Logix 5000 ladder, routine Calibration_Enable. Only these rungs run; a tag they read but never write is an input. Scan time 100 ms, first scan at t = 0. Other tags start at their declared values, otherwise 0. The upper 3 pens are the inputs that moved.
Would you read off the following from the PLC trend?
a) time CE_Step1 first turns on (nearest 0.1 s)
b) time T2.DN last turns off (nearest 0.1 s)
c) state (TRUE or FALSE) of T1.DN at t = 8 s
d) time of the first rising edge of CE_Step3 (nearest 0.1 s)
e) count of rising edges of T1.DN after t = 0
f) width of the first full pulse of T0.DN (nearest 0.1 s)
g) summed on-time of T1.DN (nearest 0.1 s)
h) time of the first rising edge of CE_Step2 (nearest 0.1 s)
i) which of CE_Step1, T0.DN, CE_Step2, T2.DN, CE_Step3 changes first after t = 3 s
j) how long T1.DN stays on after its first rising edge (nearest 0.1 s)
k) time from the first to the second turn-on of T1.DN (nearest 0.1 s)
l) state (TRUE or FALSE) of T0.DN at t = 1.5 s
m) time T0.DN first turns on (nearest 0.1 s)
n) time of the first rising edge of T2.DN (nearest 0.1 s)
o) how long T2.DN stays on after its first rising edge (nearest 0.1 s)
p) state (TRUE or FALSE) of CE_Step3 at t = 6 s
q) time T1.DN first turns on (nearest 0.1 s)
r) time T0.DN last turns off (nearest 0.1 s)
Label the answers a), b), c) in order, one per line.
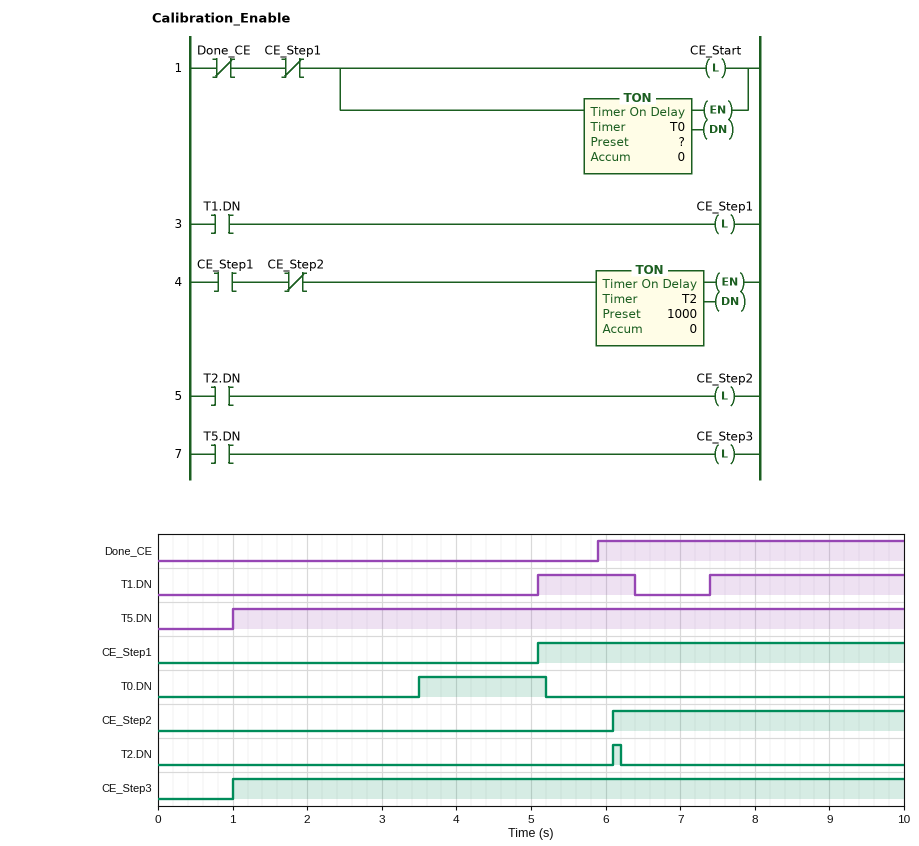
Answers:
a) 5.1 s
b) 6.2 s
c) TRUE
d) 1.0 s
e) 2
f) 1.7 s
g) 3.9 s
h) 6.1 s
i) T0.DN
j) 1.3 s
k) 2.3 s
l) FALSE
m) 3.5 s
n) 6.1 s
o) 0.1 s
p) TRUE
q) 5.1 s
r) 5.2 s
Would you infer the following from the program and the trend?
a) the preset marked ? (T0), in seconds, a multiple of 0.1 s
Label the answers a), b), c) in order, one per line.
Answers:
a) 3.5 s
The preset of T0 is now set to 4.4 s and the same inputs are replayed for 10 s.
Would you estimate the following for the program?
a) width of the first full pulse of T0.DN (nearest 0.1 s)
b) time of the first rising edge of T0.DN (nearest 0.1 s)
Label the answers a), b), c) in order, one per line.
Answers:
a) 0.8 s
b) 4.4 s
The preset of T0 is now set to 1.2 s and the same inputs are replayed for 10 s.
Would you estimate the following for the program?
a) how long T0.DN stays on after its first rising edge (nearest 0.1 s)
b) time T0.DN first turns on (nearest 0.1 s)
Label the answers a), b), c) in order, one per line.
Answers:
a) 4.0 s
b) 1.2 s
